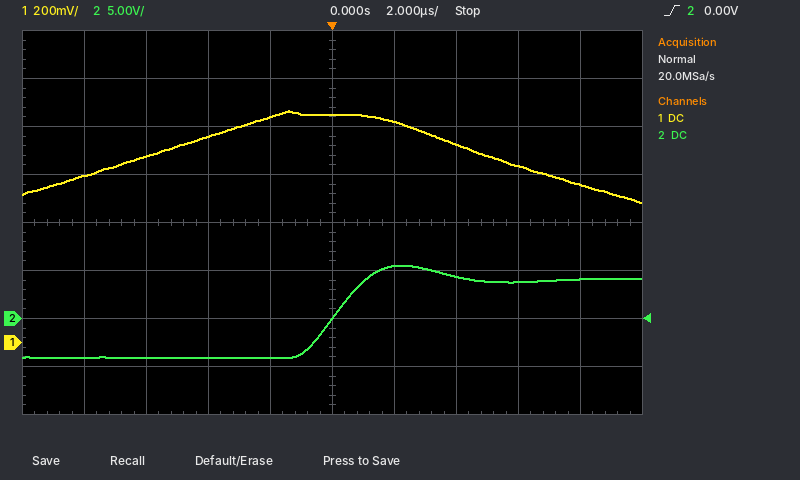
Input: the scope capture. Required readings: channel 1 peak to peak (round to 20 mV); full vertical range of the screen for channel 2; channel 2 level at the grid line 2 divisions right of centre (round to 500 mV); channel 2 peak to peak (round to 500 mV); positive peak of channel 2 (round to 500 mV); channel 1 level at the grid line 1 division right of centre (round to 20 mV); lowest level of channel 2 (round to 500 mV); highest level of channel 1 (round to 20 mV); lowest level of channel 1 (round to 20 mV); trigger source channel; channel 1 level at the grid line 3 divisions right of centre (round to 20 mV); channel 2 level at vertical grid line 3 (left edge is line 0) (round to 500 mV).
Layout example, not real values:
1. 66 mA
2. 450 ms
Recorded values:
1. 380 mV
2. 40 V
3. 4.5 V
4. 9.5 V
5. 5.5 V
6. 920 mV
7. -4.0 V
8. 960 mV
9. 580 mV
10. channel 2
11. 740 mV
12. -4.0 V
